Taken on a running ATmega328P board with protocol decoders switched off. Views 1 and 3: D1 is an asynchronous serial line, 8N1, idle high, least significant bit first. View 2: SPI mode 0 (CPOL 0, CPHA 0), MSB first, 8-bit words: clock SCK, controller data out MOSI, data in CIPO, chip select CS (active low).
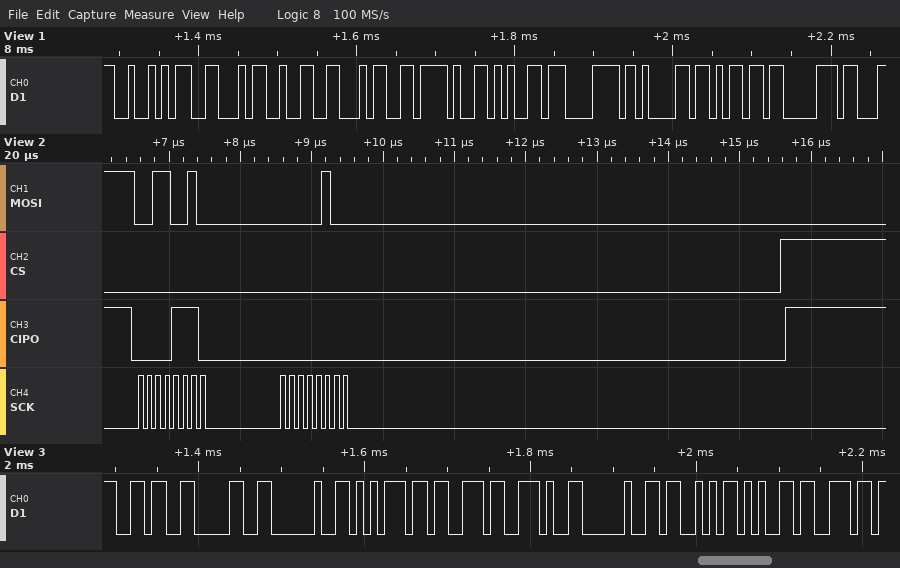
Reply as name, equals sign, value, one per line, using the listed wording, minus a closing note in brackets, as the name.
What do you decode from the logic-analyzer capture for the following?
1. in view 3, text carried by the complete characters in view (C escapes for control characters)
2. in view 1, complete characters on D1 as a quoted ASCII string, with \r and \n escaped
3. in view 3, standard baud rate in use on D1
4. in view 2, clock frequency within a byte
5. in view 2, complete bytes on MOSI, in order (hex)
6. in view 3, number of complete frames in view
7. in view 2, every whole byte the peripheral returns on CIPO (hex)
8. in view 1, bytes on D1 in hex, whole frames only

in view 3, text carried by the complete characters in view = "60 us. Sen"
in view 1, complete characters on D1 as a quoted ASCII string, with \r and \n escaped = "RF24/examp"
in view 3, standard baud rate in use on D1 = 115200 baud
in view 2, clock frequency within a byte = 8 MHz
in view 2, complete bytes on MOSI, in order = 32 04
in view 3, number of complete frames in view = 10
in view 2, every whole byte the peripheral returns on CIPO = 0E 00
in view 1, bytes on D1 in hex, whole frames only = 52 46 32 34 2F 65 78 61 6D 70
